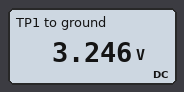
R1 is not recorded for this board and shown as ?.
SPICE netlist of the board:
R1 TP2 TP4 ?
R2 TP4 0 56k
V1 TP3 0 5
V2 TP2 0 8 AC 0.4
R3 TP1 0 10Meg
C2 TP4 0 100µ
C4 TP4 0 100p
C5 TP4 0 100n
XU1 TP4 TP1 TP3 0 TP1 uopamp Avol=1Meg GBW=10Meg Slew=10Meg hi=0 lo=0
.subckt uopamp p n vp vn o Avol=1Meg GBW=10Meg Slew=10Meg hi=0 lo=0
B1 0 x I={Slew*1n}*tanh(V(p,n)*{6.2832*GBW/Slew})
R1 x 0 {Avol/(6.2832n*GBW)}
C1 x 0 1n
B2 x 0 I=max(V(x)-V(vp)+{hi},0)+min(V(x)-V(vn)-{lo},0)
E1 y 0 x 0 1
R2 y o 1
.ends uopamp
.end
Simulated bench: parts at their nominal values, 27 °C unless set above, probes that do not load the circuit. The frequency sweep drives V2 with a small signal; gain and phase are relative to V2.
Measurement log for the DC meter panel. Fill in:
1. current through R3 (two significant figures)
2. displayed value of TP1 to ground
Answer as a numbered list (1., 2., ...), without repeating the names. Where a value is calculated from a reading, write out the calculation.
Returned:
1. (3.246 V) / 10 MΩ = 320 nA
2. 3.246 V
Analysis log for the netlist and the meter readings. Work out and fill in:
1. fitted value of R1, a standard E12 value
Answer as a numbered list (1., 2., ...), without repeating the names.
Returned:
1. 82 kΩ
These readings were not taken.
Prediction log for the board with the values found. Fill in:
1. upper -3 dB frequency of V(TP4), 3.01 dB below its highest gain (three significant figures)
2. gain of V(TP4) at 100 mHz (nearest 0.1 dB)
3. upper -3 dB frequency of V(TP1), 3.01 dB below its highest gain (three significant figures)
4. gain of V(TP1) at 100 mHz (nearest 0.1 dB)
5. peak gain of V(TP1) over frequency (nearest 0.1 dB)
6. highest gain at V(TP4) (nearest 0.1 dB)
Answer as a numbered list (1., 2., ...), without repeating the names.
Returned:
1. 47.8 mHz
2. -15.1 dB
3. 47.8 mHz
4. -15.1 dB
5. -7.8 dB
6. -7.8 dB
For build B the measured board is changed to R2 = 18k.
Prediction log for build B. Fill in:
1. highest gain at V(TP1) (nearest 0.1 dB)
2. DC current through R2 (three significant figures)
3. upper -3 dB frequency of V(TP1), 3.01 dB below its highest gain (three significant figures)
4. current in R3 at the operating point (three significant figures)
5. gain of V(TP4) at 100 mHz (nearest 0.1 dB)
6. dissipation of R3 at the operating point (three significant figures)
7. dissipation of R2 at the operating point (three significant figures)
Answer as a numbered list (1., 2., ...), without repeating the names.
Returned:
1. -14.9 dB
2. 80.0 µA
3. 108 mHz
4. 144 nA
5. -17.6 dB
6. 207 nW
7. 115 µW
